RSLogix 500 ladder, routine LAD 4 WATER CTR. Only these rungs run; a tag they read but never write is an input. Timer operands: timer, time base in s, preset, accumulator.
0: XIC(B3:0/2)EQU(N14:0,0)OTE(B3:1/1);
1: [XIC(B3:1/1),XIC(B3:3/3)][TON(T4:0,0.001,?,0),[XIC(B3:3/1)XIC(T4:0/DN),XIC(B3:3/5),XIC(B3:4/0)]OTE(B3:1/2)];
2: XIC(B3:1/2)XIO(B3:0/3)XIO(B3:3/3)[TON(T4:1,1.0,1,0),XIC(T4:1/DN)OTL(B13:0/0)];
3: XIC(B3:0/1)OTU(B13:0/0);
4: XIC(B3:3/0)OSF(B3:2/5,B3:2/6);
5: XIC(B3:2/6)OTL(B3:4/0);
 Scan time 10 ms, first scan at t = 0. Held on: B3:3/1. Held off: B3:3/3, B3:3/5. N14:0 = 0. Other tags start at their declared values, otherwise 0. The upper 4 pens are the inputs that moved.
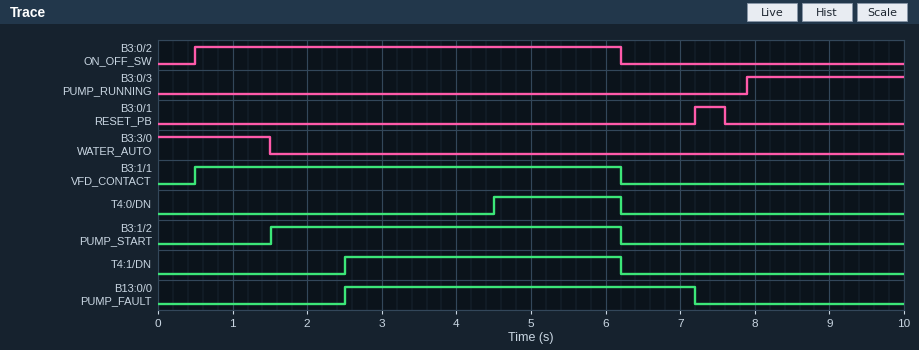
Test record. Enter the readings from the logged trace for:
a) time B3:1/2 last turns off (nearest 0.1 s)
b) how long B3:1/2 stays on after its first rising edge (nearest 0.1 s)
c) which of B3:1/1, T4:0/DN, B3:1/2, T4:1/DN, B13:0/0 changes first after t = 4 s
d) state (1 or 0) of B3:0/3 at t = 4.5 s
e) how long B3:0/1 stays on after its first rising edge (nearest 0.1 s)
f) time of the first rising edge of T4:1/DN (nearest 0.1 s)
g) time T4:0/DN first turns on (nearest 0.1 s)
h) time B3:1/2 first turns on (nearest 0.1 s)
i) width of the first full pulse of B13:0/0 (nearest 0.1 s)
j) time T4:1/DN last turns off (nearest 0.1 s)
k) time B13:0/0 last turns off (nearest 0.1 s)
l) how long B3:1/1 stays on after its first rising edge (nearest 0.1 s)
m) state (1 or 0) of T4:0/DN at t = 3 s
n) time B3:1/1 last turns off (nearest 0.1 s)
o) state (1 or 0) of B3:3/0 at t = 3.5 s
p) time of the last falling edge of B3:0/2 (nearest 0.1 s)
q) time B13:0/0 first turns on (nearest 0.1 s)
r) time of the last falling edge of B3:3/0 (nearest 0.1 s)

6.2 s
4.7 s
T4:0/DN
0
0.4 s
2.5 s
4.5 s
1.5 s
4.7 s
6.2 s
7.2 s
5.7 s
0
6.2 s
0
6.2 s
2.5 s
1.5 s
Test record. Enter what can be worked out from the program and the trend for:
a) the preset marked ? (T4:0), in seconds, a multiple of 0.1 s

4.0 s
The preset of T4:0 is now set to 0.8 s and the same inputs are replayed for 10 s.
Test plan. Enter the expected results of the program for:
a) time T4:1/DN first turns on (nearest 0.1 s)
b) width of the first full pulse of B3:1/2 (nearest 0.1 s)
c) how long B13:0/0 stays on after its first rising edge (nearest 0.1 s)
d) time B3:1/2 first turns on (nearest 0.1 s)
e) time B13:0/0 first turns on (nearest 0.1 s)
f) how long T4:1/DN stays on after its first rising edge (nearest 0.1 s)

2.3 s
4.9 s
4.9 s
1.3 s
2.3 s
3.9 s
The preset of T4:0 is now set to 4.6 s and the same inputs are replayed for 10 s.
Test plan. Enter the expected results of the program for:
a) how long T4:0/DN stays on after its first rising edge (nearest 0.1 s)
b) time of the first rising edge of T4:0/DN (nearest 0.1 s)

1.1 s
5.1 s
